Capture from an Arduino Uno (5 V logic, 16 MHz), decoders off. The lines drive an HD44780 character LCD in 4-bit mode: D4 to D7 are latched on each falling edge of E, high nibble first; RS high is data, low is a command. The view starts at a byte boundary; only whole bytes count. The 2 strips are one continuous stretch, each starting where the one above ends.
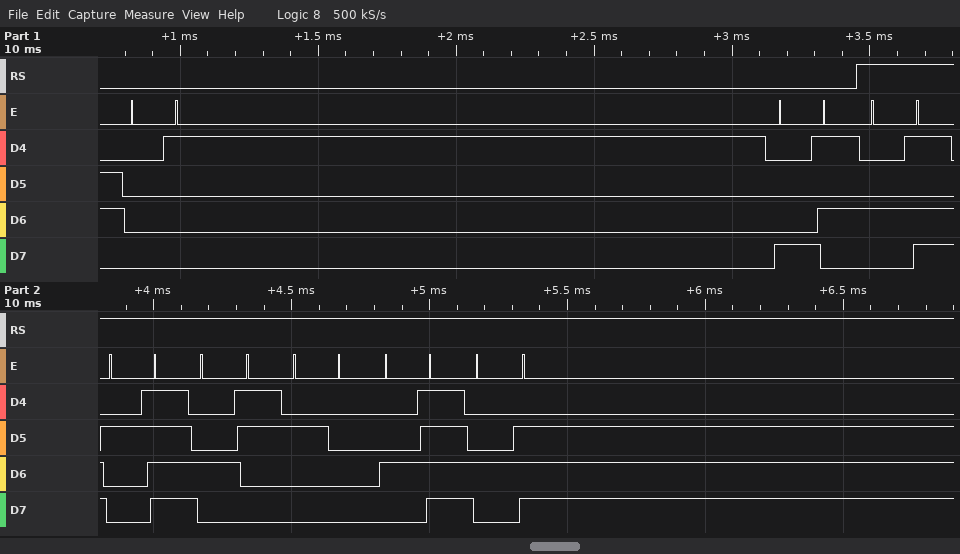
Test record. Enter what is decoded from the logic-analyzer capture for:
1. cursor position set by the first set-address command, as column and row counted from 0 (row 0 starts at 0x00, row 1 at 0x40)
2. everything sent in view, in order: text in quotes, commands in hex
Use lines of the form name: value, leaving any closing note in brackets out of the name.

cursor position set by the first set-address command, as column and row counted from 0: column 5, row 0
everything sent in view, in order: text in quotes, commands in hex: 0x01 0x85 "M/C ON"
